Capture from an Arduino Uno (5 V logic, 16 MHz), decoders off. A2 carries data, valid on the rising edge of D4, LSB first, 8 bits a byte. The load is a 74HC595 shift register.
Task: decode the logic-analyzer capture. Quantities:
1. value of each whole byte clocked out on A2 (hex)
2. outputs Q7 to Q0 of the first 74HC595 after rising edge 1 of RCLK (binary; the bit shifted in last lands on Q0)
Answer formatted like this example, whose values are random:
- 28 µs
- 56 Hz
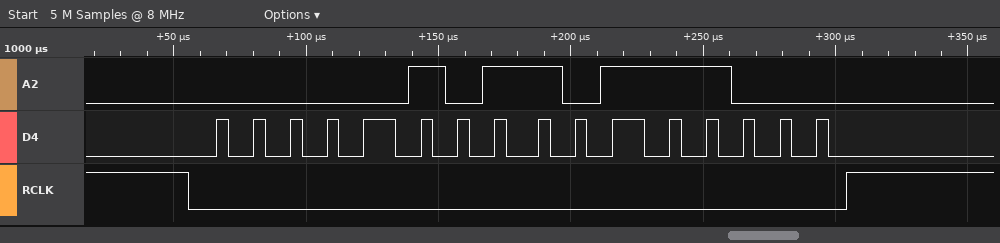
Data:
- 0xA0 0x1D
- 10111000
